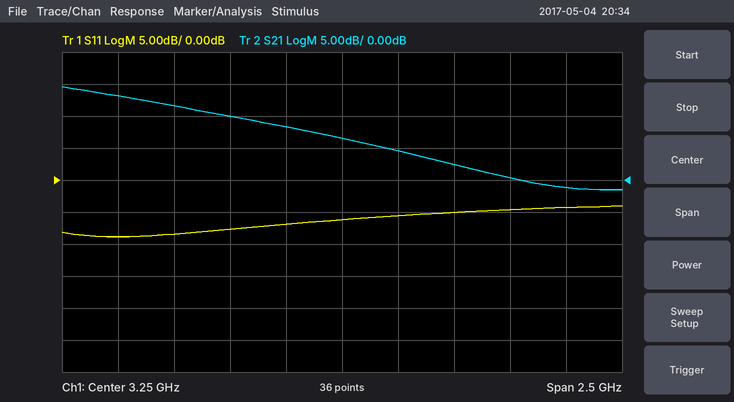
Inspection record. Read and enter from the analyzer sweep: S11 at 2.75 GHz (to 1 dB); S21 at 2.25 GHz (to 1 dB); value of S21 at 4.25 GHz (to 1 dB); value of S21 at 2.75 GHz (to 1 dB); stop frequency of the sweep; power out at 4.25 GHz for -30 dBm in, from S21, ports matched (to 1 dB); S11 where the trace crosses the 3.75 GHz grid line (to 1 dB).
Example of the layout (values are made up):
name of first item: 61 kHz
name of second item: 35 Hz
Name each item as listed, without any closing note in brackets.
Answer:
S11 at 2.75 GHz: -8 dB
S21 at 2.25 GHz: 13 dB
value of S21 at 4.25 GHz: -1 dB
value of S21 at 2.75 GHz: 10 dB
stop frequency of the sweep: 4.5 GHz
power out at 4.25 GHz for -30 dBm in, from S21, ports matched: -31 dBm
S11 where the trace crosses the 3.75 GHz grid line: -5 dB
